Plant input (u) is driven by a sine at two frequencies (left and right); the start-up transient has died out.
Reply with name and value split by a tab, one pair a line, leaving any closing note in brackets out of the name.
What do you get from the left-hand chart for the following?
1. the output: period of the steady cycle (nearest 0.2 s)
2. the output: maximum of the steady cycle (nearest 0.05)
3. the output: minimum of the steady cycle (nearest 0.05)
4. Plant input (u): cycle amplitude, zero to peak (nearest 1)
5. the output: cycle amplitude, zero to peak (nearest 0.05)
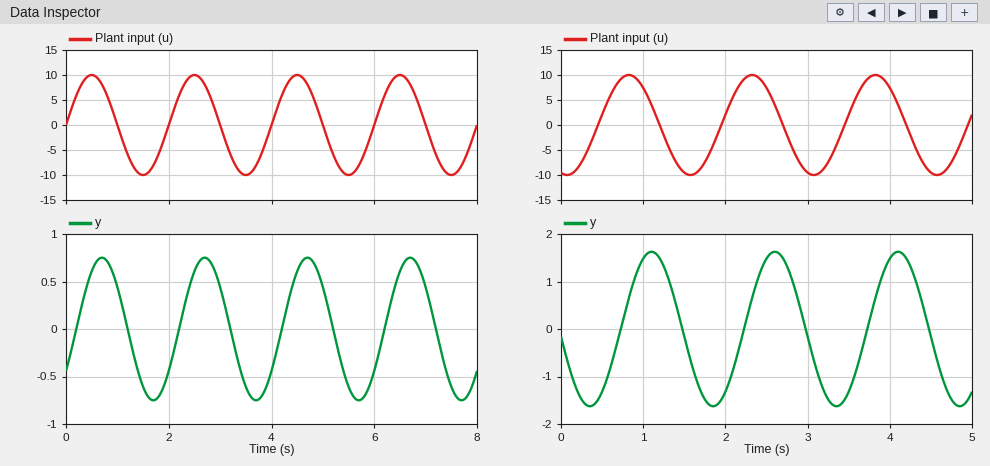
the output: period of the steady cycle	2.0 s
the output: maximum of the steady cycle	0.75
the output: minimum of the steady cycle	-0.75
Plant input (u): cycle amplitude, zero to peak	10
the output: cycle amplitude, zero to peak	0.75
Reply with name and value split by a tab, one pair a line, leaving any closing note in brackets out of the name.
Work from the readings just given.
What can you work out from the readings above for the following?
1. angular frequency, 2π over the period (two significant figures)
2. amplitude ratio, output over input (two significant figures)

angular frequency, 2π over the period	3.1 rad/s
amplitude ratio, output over input	0.075
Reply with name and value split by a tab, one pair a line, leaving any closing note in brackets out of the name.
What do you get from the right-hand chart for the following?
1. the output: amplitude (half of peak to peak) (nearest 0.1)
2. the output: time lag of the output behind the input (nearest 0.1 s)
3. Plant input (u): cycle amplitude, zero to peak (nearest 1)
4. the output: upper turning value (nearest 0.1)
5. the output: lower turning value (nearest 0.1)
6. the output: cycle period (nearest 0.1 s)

the output: amplitude (half of peak to peak)	1.6
the output: time lag of the output behind the input	0.3 s
Plant input (u): cycle amplitude, zero to peak	10
the output: upper turning value	1.6
the output: lower turning value	-1.6
the output: cycle period	1.5 s
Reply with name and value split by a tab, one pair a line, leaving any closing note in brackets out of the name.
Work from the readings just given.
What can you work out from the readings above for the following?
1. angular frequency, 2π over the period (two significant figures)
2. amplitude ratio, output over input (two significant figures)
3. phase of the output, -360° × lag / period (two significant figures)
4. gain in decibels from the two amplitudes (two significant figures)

angular frequency, 2π over the period	4.2 rad/s
amplitude ratio, output over input	0.16
phase of the output, -360° × lag / period	-72°
gain in decibels from the two amplitudes	-16 dB
